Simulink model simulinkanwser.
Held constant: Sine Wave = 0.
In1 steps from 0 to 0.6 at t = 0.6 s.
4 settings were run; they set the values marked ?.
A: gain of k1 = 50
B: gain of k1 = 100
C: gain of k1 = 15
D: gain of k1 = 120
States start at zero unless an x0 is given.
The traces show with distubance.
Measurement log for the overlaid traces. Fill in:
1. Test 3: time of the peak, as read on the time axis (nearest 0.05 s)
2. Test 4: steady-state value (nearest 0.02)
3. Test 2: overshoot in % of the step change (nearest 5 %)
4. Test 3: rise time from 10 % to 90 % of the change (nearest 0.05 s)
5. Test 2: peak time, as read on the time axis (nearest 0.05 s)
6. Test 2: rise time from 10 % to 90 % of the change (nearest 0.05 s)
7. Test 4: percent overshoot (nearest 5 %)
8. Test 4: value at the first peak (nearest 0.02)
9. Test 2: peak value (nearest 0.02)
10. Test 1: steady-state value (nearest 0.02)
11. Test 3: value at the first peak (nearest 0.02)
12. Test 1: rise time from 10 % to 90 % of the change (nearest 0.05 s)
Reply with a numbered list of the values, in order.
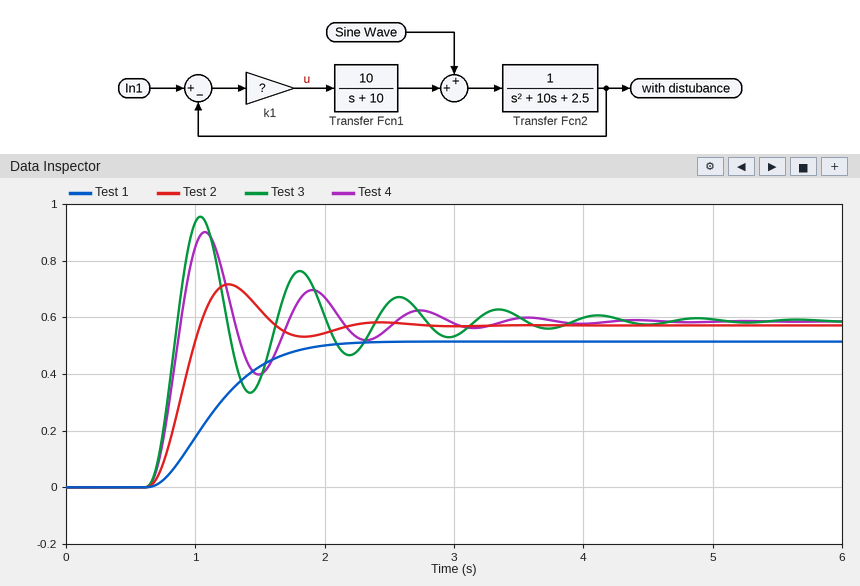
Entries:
1. 1.05 s
2. 0.58
3. 25 %
4. 0.15 s
5. 1.25 s
6. 0.25 s
7. 55 %
8. 0.90
9. 0.72
10. 0.52
11. 0.96
12. 0.85 s
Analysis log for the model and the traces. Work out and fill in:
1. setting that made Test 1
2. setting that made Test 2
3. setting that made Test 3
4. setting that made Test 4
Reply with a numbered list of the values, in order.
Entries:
1. C
2. A
3. D
4. B
